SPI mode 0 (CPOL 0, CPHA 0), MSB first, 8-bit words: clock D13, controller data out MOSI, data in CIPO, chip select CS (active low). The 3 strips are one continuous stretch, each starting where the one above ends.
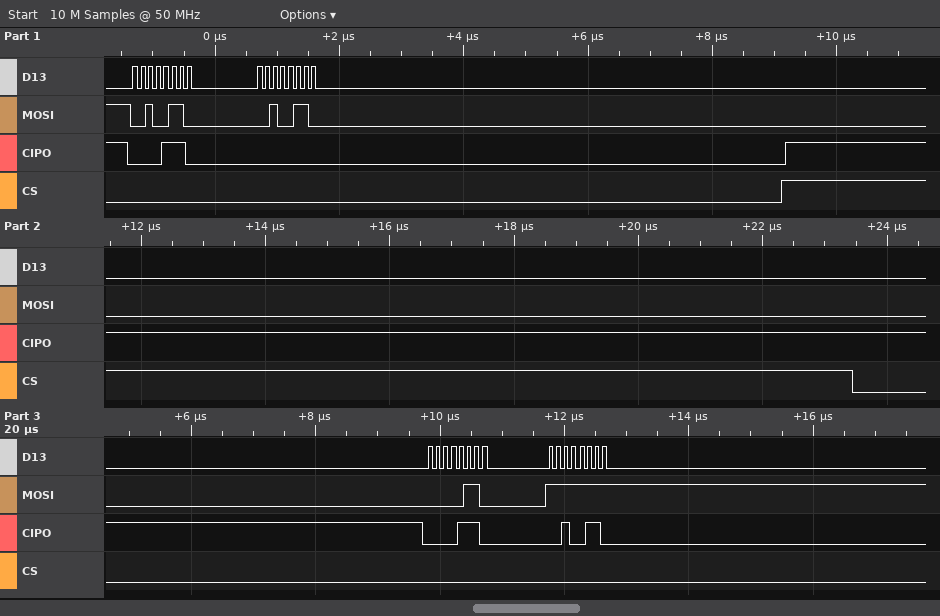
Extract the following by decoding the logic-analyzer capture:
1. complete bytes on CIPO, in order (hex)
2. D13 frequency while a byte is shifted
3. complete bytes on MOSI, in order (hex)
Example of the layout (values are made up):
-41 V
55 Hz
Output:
0E 00 0E 26
8 MHz
26 26 06 FF
